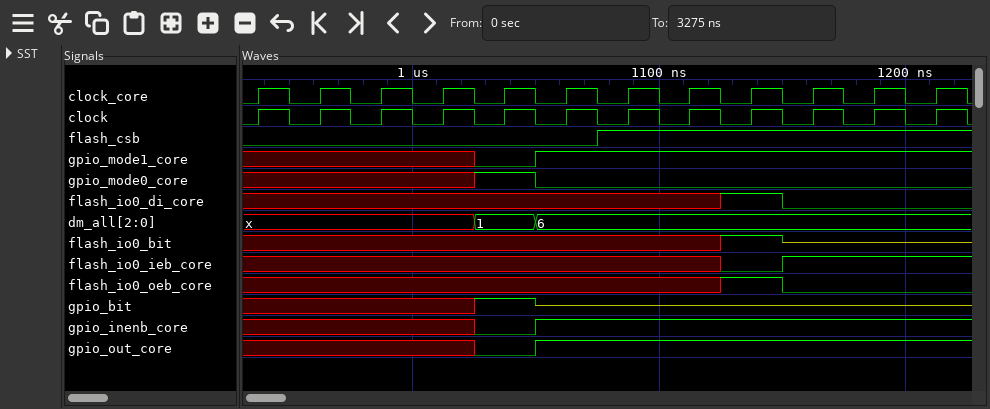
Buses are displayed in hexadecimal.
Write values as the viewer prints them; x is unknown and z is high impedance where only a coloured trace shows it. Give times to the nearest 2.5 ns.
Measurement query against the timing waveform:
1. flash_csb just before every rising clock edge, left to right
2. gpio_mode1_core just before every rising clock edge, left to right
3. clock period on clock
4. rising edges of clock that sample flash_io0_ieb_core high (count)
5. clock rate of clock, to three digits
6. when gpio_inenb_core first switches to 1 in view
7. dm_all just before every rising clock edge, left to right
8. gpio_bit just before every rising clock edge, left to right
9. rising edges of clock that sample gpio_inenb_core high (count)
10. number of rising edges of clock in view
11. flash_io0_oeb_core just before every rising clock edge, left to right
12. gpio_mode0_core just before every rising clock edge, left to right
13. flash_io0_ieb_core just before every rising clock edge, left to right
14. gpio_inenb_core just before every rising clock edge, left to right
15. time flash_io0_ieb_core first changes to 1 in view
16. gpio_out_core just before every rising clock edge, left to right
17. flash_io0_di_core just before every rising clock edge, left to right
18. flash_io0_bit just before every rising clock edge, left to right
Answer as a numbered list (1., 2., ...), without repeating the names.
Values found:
1. 0 0 0 0 0 0 1 1 1 1 1 1
2. x x x x 0 1 1 1 1 1 1 1
3. 25 ns
4. 3
5. 40.0 MHz
6. 1050 ns
7. x, x, x, x, 1, 6, 6, 6, 6, 6, 6, 6
8. x x x x 1 z z z z z z z
9. 7
10. 12
11. x x x x x x x x 1 0 0 0
12. x x x x 1 0 0 0 0 0 0 0
13. x x x x x x x x 0 1 1 1
14. x x x x 0 1 1 1 1 1 1 1
15. 1150 ns
16. x x x x 0 1 1 1 1 1 1 1
17. x x x x x x x x 1 0 0 0
18. x x x x x x x x 1 z z z
